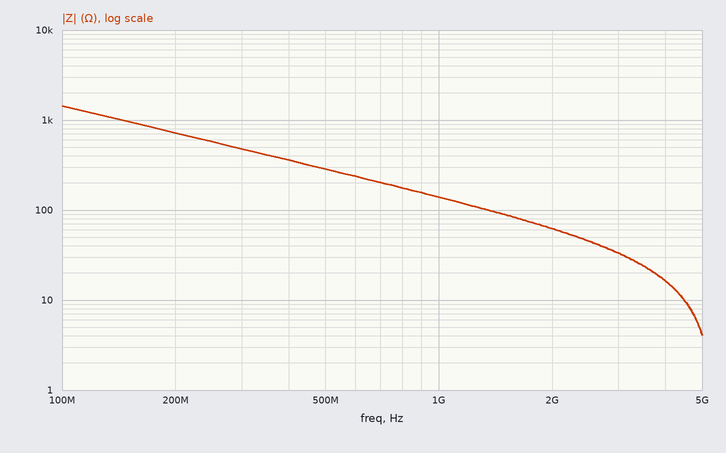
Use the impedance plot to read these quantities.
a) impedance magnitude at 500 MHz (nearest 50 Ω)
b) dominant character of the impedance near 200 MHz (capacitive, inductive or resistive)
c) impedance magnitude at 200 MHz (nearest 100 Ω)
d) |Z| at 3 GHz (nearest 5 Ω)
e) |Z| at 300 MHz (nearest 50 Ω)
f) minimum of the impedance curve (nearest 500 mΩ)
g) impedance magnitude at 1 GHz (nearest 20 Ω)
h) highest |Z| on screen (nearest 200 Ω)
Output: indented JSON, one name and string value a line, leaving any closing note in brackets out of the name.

{
  "impedance magnitude at 500 MHz": "300 Ω",
  "dominant character of the impedance near 200 MHz": "capacitive",
  "impedance magnitude at 200 MHz": "700 Ω",
  "|Z| at 3 GHz": "35 Ω",
  "|Z| at 300 MHz": "500 Ω",
  "minimum of the impedance curve": "4.0 Ω",
  "impedance magnitude at 1 GHz": "140 Ω",
  "highest |Z| on screen": "1.4 kΩ"
}
